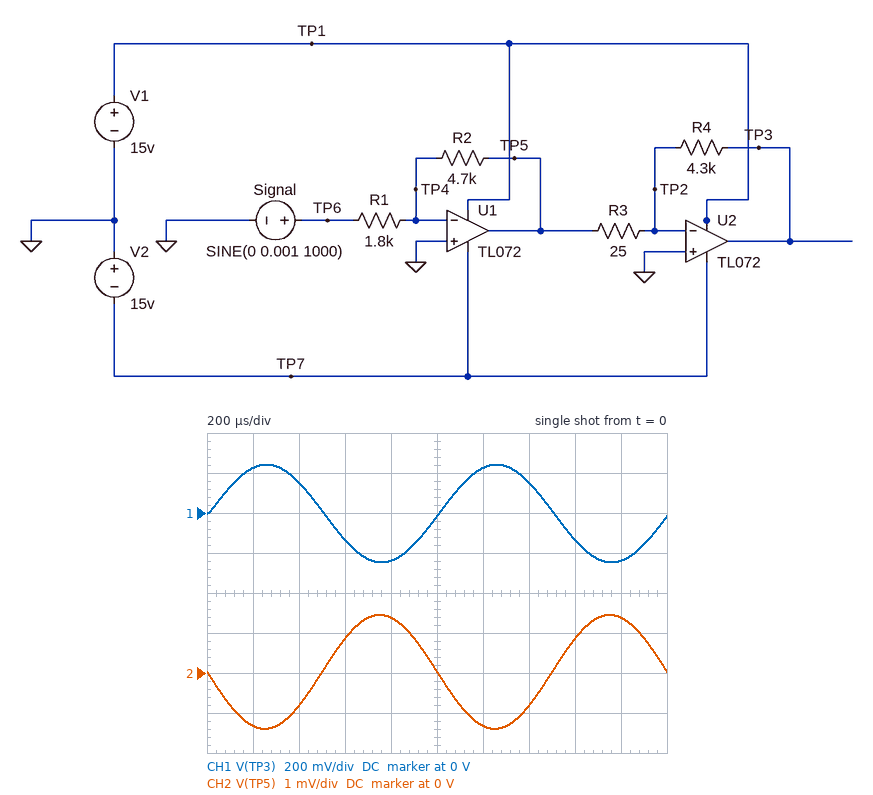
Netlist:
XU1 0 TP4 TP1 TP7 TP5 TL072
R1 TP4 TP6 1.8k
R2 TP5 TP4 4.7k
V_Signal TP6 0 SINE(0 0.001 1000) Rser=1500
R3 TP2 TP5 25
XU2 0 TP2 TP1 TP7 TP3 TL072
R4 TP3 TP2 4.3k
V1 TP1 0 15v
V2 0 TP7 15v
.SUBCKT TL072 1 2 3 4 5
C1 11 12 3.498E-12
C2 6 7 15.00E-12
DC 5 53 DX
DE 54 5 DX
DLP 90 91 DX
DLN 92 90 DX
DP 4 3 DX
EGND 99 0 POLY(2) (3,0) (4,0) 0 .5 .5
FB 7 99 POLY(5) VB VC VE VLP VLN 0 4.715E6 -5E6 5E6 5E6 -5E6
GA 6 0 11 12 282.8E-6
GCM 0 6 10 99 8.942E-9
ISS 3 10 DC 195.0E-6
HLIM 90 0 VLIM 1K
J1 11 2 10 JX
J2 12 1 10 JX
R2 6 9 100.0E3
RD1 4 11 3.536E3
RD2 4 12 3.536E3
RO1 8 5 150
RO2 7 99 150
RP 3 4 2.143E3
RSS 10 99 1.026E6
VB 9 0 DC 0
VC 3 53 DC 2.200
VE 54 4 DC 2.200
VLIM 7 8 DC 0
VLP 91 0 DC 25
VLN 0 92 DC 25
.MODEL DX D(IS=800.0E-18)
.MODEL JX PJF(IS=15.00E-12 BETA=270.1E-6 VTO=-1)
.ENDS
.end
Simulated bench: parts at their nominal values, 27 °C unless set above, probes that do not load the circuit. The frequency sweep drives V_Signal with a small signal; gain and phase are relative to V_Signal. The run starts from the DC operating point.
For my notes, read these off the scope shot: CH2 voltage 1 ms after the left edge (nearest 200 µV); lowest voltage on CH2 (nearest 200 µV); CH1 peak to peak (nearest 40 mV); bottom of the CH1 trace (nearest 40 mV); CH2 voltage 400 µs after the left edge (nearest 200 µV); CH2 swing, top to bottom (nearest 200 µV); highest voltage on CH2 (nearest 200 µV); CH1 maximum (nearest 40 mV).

0 V
-1.4 mV
480 mV
-240 mV
-800 µV
2.8 mV
1.4 mV
240 mV
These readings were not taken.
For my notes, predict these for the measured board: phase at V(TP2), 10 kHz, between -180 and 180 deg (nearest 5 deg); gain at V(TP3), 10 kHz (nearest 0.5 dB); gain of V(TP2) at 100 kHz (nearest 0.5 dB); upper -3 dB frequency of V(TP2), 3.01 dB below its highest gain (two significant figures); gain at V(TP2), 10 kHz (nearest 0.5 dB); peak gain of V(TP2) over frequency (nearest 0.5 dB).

-120 deg
46.5 dB
2.0 dB
1.9 MHz
-4.0 dB
2.5 dB
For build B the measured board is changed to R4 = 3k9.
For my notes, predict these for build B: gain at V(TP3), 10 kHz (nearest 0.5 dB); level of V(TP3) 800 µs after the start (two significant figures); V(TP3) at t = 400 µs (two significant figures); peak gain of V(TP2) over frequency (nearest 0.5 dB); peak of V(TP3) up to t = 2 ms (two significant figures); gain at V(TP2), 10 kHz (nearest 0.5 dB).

46.0 dB
-220 mV
140 mV
2.0 dB
220 mV
-4.5 dB
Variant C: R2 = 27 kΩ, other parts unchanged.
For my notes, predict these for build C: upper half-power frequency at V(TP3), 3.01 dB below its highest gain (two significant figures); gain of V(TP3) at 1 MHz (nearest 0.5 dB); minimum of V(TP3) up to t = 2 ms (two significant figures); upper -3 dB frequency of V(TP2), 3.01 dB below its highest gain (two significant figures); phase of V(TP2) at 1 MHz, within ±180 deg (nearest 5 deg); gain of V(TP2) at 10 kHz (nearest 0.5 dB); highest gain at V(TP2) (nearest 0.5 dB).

15 kHz
19.5 dB
-1.4 V
540 kHz
110 deg
11.0 dB
15.5 dB
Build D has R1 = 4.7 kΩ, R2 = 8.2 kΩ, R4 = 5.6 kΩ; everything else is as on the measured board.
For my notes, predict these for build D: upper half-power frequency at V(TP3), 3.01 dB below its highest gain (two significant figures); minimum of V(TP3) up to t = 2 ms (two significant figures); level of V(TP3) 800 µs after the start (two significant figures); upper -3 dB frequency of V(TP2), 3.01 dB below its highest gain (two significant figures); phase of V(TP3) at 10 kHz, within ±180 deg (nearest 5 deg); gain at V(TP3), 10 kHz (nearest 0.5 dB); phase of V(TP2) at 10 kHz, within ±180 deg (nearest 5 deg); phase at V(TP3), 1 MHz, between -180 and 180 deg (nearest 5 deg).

14 kHz
-300 mV
-290 mV
2.0 MHz
-35 deg
47.5 dB
-125 deg
-135 deg
